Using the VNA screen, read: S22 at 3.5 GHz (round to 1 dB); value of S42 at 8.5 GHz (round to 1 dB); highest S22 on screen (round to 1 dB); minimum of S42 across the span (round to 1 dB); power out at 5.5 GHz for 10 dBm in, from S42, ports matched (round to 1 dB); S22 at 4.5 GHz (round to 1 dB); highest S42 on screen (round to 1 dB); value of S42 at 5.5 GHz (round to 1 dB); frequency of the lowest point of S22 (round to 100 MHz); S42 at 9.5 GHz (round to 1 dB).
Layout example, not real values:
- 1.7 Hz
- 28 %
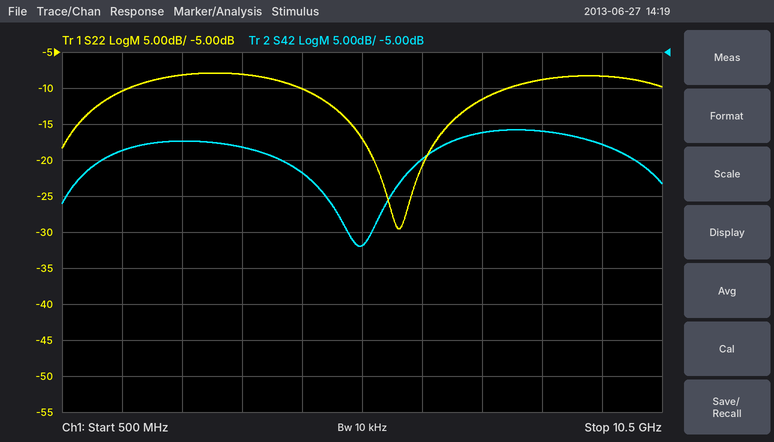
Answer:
- -8 dB
- -16 dB
- -8 dB
- -32 dB
- -22 dBm
- -10 dB
- -16 dB
- -32 dB
- 6.1 GHz
- -18 dB
